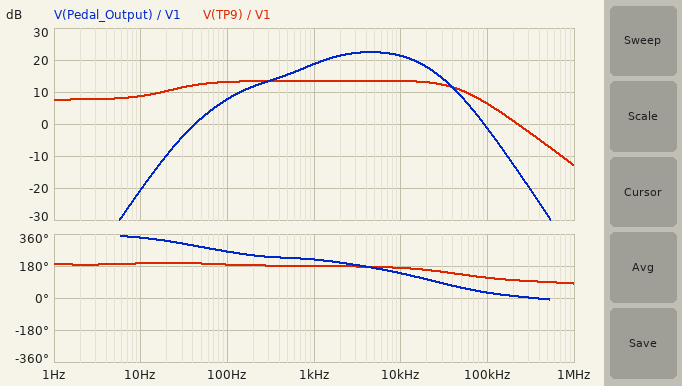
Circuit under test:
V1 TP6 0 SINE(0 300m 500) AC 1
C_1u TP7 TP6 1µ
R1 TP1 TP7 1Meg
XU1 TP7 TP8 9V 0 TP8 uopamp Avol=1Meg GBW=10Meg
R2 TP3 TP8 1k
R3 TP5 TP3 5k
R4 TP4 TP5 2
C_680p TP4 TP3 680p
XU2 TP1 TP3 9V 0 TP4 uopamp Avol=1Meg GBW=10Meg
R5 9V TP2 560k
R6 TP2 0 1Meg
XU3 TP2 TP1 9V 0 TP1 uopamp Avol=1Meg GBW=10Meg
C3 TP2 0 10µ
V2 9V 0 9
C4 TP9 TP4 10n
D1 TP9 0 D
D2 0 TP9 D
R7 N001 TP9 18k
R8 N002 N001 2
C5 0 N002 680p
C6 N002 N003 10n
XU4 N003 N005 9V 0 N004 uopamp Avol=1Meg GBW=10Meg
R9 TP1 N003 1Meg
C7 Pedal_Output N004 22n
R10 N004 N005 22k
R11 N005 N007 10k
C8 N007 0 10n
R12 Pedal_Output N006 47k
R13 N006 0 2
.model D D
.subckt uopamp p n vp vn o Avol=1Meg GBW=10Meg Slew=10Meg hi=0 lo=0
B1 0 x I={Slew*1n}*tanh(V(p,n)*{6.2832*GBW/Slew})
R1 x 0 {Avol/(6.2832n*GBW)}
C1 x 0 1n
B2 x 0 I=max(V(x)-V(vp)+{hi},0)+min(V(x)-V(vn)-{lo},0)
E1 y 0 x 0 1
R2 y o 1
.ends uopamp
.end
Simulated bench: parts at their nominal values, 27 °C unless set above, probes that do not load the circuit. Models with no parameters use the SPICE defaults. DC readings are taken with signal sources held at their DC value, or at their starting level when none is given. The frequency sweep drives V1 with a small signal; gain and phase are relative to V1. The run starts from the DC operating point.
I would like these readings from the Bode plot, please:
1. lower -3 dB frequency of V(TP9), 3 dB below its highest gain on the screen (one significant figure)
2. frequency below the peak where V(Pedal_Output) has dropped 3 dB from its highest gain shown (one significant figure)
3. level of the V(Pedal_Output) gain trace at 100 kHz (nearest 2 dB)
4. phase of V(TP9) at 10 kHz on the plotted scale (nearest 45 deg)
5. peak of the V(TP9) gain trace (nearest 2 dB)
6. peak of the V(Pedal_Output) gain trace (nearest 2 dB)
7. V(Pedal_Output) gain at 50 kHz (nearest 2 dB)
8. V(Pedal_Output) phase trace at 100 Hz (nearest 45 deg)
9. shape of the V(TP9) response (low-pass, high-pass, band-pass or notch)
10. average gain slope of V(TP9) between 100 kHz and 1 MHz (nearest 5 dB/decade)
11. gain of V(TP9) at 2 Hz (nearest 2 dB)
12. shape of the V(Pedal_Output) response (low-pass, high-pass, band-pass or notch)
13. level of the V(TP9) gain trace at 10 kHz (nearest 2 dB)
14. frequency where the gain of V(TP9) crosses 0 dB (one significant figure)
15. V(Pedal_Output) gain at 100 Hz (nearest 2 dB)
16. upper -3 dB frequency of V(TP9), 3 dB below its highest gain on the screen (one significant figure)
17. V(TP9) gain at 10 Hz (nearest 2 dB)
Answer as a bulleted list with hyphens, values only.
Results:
- 20 Hz
- 1 kHz
- -2 dB
- 180 deg
- 14 dB
- 22 dB
- 8 dB
- 270 deg
- low-pass
- -20 dB/decade
- 8 dB
- band-pass
- 14 dB
- 200 kHz
- 8 dB
- 50 kHz
- 8 dB
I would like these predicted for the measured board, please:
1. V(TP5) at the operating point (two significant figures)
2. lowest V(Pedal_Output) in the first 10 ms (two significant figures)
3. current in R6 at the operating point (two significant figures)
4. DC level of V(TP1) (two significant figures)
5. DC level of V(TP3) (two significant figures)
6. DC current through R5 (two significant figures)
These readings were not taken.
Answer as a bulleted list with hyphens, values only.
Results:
- 5.8 V
- -1.3 V
- 5.8 µA
- 5.8 V
- 5.8 V
- 5.8 µA
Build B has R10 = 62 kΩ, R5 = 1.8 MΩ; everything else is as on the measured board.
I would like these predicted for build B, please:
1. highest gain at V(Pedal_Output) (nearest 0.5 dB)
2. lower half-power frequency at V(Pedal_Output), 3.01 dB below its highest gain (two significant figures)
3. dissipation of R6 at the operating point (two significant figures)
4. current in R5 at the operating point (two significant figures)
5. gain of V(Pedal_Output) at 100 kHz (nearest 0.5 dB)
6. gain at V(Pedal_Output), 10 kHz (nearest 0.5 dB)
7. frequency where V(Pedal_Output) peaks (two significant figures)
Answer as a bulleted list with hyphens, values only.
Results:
- 29.5 dB
- 1.3 kHz
- 10 µW
- 3.2 µA
- 5.5 dB
- 28.5 dB
- 4.6 kHz
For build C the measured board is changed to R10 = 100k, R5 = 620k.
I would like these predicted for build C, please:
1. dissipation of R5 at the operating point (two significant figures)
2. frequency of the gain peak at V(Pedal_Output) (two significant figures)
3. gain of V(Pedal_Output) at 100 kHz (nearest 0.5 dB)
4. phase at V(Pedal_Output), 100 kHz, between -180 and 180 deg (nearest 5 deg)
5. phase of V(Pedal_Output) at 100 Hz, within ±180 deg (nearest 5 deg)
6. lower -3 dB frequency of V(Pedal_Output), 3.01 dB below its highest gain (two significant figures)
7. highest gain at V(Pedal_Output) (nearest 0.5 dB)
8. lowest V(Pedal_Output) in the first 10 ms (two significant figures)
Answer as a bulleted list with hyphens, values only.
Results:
- 19 µW
- 4.6 kHz
- 9.5 dB
- 25 deg
- -75 deg
- 1.3 kHz
- 33.0 dB
- -3.7 V
